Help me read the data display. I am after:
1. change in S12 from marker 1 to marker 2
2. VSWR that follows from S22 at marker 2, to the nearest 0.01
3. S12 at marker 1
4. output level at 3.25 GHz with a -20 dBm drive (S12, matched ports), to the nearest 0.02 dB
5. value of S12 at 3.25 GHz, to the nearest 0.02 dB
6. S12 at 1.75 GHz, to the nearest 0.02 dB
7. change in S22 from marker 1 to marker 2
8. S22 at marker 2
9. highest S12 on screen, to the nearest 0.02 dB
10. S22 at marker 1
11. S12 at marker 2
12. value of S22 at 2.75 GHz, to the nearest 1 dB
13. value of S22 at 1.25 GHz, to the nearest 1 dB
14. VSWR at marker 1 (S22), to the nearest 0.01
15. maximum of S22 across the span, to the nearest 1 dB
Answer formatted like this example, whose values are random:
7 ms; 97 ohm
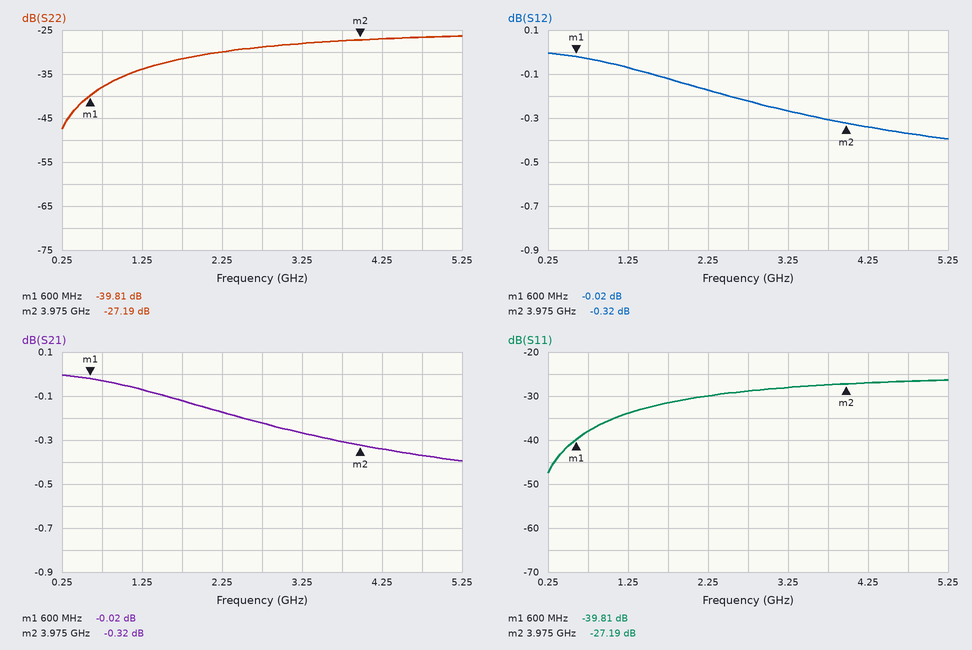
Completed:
-0.30 dB; 1.09; -0.02 dB; -20.26 dBm; -0.26 dB; -0.12 dB; 12.62 dB; -27.19 dB; 0.00 dB; -39.81 dB; -0.32 dB; -29 dB; -34 dB; 1.02; -26 dB
